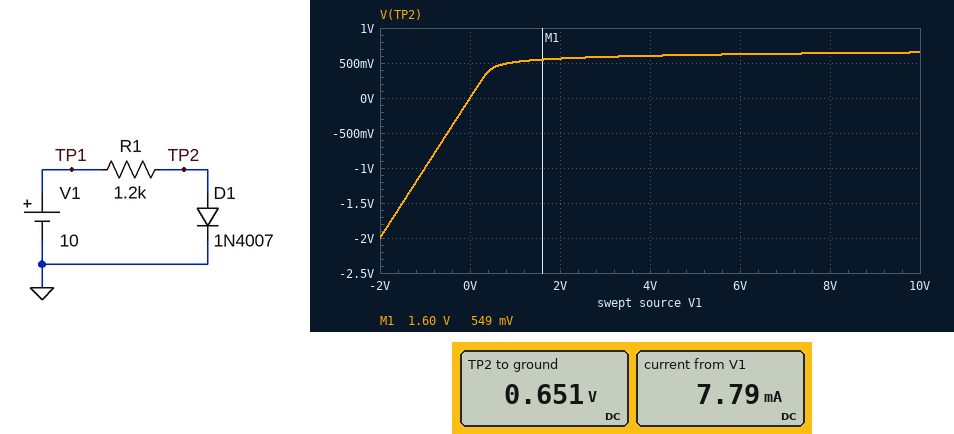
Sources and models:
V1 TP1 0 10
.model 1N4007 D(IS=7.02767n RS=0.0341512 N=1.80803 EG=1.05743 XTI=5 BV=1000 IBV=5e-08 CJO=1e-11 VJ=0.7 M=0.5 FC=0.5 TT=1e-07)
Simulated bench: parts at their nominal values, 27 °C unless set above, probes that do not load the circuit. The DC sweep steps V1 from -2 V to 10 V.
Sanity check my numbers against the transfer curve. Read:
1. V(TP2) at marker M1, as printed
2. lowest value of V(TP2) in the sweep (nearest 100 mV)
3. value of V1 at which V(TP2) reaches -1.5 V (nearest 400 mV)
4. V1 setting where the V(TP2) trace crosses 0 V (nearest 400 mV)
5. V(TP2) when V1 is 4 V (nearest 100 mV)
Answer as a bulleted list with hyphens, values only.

- 549 mV
- -2.0 V
- -1.6 V
- 0 V
- 600 mV
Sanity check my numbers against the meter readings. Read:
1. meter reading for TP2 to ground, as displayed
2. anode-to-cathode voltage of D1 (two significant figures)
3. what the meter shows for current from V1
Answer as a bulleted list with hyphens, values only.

- 0.651 V
- 650 mV
- 7.79 mA
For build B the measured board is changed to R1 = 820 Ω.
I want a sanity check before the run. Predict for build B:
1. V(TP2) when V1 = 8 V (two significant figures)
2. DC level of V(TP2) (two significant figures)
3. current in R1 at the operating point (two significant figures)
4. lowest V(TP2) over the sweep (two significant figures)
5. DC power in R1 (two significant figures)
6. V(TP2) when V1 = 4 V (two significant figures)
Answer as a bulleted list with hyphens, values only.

- 660 mV
- 670 mV
- 11 mA
- -2.0 V
- 110 mW
- 620 mV
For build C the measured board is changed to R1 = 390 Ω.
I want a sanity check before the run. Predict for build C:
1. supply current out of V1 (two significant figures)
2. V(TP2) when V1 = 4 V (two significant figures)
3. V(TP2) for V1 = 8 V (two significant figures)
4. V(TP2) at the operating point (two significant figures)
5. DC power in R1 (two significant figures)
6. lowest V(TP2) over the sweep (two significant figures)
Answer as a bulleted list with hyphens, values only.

- 24 mA
- 660 mV
- 690 mV
- 700 mV
- 220 mW
- -2.0 V
